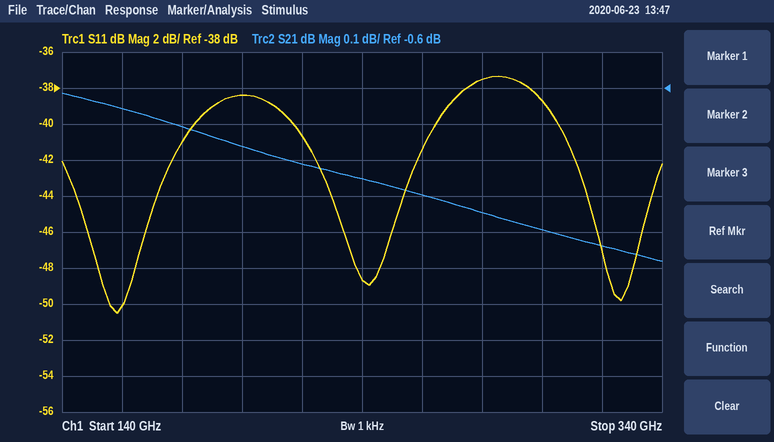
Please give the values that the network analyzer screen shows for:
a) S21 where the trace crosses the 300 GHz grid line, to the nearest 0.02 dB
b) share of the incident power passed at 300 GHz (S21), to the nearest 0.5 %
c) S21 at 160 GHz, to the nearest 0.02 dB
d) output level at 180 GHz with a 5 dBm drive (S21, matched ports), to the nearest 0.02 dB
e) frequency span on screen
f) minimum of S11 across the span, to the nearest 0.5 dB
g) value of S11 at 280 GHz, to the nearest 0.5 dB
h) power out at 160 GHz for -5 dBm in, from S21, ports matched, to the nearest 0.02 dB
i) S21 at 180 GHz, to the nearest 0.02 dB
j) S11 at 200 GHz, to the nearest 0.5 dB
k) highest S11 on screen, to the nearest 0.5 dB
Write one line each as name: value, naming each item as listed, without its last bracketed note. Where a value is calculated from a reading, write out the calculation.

S21 where the trace crosses the 300 GHz grid line, to the nearest 0.02 dB: -1.00 dB
share of the incident power passed at 300 GHz (S21), to the nearest 0.5 %: 10^(-1/10) ≈ 79.4 %, so 79.5 % to the nearest 0.5 %
S21 at 160 GHz, to the nearest 0.02 dB: -0.66 dB
output level at 180 GHz with a 5 dBm drive (S21, matched ports), to the nearest 0.02 dB: 5 dBm + (-0.70 dB) = 4.30 dBm
frequency span on screen: 200 GHz
minimum of S11 across the span, to the nearest 0.5 dB: -50.5 dB
value of S11 at 280 GHz, to the nearest 0.5 dB: -37.5 dB
power out at 160 GHz for -5 dBm in, from S21, ports matched, to the nearest 0.02 dB: -5 dBm + (-0.66 dB) = -5.66 dBm
S21 at 180 GHz, to the nearest 0.02 dB: -0.70 dB
S11 at 200 GHz, to the nearest 0.5 dB: -38.5 dB
highest S11 on screen, to the nearest 0.5 dB: -37.5 dB
